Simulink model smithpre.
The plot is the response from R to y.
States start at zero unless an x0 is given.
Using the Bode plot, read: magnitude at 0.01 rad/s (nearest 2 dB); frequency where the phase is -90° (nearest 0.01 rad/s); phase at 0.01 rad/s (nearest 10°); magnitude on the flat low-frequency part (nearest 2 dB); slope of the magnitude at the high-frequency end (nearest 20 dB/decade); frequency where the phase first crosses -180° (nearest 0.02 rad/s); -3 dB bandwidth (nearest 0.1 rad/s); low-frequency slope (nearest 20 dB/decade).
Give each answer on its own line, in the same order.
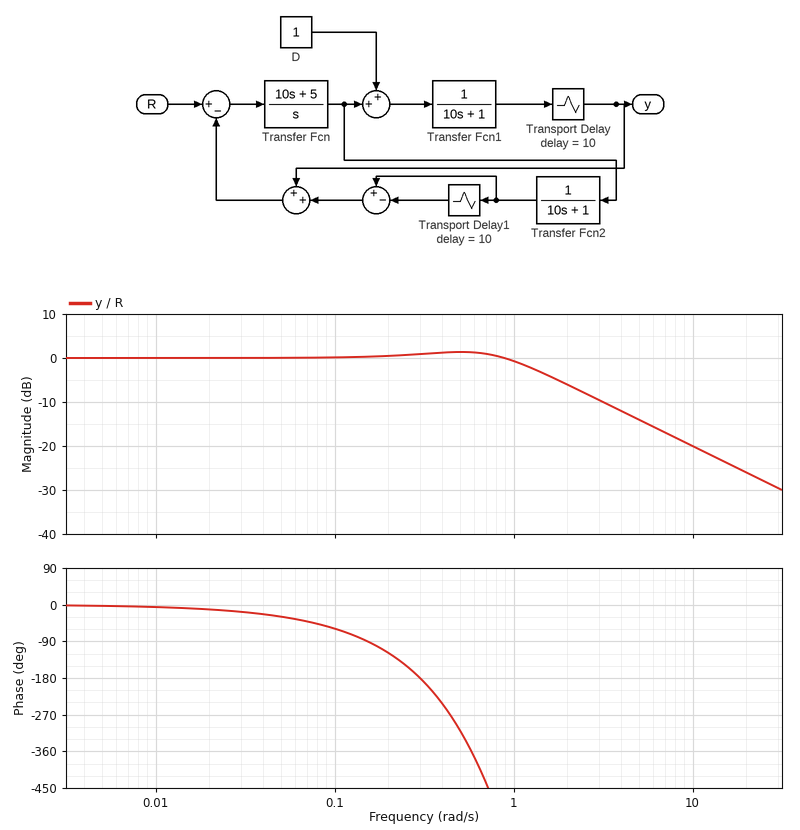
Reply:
0 dB
0.15 rad/s
-10°
0 dB
-20 dB/decade
0.30 rad/s
1.4 rad/s
0 dB/decade
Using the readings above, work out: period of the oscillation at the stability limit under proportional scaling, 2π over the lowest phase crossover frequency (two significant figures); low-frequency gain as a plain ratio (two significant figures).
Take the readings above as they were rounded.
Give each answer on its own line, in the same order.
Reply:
21 s
1.0
